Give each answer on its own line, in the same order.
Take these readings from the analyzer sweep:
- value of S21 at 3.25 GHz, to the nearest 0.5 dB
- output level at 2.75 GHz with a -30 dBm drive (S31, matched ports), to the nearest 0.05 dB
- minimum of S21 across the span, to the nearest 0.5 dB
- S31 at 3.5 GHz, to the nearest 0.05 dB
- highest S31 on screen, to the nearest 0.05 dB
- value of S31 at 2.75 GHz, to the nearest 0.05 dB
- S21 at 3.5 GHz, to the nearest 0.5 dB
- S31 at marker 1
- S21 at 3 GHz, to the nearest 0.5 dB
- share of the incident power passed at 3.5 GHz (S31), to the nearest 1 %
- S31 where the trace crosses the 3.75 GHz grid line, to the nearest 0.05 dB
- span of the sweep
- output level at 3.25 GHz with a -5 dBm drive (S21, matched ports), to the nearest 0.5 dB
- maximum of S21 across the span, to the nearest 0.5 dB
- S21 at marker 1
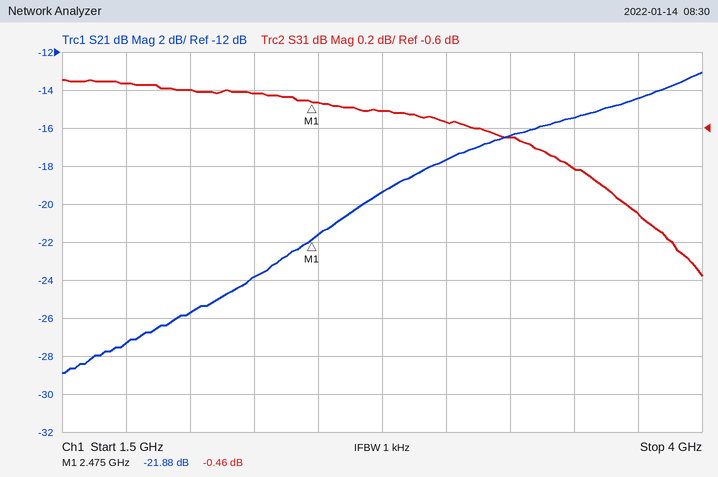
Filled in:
-16.5 dB
-30.50 dBm
-29.0 dB
-0.80 dB
-0.35 dB
-0.50 dB
-15.5 dB
-0.46 dB
-17.5 dB
83 %
-1.05 dB
2.5 GHz
-21.5 dBm
-13.0 dB
-21.88 dB
